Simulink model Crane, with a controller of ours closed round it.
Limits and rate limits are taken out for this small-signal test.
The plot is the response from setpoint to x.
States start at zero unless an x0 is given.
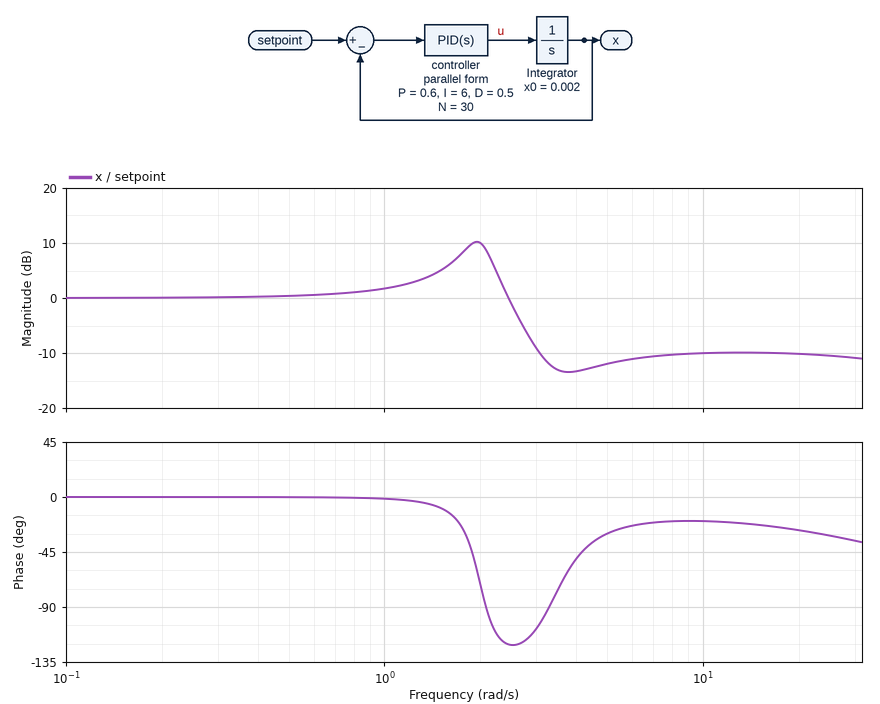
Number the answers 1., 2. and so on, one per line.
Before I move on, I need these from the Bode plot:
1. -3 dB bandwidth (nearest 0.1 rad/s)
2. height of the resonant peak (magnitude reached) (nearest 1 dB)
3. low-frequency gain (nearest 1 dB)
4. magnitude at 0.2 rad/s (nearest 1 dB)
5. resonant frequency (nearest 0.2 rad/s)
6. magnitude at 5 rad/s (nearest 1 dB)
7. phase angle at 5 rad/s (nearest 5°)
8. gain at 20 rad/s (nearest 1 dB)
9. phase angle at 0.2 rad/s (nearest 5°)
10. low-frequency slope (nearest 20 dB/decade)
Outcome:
1. 2.6 rad/s
2. 10 dB
3. 0 dB
4. 0 dB
5. 2.0 rad/s
6. -12 dB
7. -30°
8. -10 dB
9. 0°
10. 0 dB/decade
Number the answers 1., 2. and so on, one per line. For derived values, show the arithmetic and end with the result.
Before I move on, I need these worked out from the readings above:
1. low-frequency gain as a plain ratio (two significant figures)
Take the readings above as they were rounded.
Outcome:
1. 10^(0 / 20) = 1.0
